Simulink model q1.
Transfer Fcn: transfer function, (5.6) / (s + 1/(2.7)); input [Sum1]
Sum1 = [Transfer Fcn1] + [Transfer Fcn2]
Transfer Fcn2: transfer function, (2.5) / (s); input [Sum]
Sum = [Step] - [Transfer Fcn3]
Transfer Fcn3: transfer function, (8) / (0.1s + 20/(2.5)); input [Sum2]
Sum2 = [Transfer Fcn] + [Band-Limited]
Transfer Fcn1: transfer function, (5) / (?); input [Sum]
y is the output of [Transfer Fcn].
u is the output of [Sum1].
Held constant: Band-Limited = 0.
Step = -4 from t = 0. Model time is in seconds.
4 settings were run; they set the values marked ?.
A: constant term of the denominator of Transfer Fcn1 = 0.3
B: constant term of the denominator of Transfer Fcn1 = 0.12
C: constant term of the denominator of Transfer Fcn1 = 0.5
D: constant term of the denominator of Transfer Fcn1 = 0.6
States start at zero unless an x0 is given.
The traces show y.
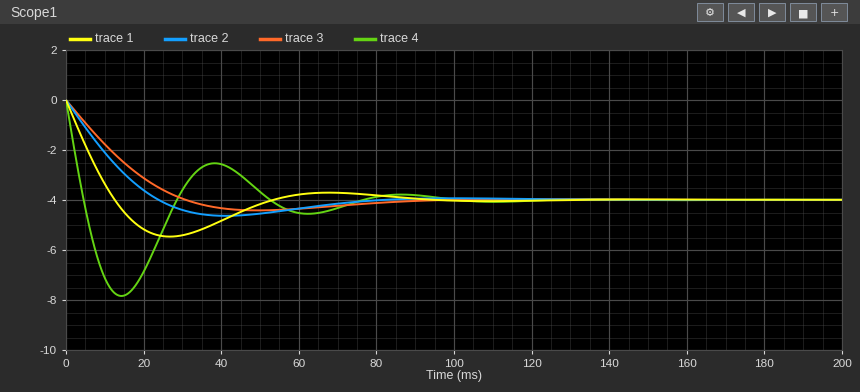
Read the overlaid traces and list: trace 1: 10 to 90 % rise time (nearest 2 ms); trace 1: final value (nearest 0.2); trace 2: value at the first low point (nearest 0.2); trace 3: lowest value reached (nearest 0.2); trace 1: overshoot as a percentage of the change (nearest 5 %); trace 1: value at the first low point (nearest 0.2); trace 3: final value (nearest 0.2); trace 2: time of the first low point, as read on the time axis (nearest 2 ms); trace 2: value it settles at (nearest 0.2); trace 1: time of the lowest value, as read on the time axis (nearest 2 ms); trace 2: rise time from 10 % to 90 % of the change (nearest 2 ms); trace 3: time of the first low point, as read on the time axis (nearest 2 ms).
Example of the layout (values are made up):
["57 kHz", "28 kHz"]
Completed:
["10 ms", "-4.0", "-4.6", "-4.4", "35 %", "-5.4", "-4.0", "42 ms", "-4.0", "26 ms", "18 ms", "50 ms"]
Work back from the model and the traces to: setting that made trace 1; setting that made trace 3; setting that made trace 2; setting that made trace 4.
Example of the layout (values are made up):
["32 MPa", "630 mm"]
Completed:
["A", "D", "C", "B"]
